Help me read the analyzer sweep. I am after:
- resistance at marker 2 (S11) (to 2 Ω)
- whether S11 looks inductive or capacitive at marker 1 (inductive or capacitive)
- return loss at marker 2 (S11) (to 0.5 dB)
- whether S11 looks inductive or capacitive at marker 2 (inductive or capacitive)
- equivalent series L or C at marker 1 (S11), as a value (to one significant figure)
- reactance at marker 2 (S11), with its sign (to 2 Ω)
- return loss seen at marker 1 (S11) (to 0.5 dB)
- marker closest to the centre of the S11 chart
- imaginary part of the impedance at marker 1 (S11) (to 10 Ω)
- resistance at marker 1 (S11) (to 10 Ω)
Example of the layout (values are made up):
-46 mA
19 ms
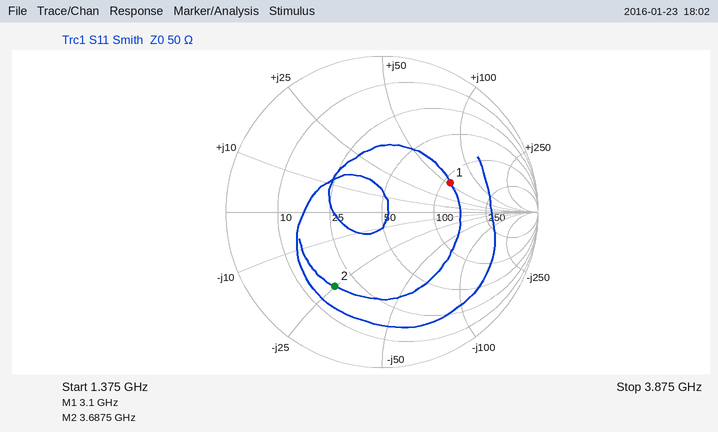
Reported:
18 Ω
inductive
5.0 dB
capacitive
3 nH
-24 Ω
6.5 dB
marker 1
+50 Ω
110 Ω
